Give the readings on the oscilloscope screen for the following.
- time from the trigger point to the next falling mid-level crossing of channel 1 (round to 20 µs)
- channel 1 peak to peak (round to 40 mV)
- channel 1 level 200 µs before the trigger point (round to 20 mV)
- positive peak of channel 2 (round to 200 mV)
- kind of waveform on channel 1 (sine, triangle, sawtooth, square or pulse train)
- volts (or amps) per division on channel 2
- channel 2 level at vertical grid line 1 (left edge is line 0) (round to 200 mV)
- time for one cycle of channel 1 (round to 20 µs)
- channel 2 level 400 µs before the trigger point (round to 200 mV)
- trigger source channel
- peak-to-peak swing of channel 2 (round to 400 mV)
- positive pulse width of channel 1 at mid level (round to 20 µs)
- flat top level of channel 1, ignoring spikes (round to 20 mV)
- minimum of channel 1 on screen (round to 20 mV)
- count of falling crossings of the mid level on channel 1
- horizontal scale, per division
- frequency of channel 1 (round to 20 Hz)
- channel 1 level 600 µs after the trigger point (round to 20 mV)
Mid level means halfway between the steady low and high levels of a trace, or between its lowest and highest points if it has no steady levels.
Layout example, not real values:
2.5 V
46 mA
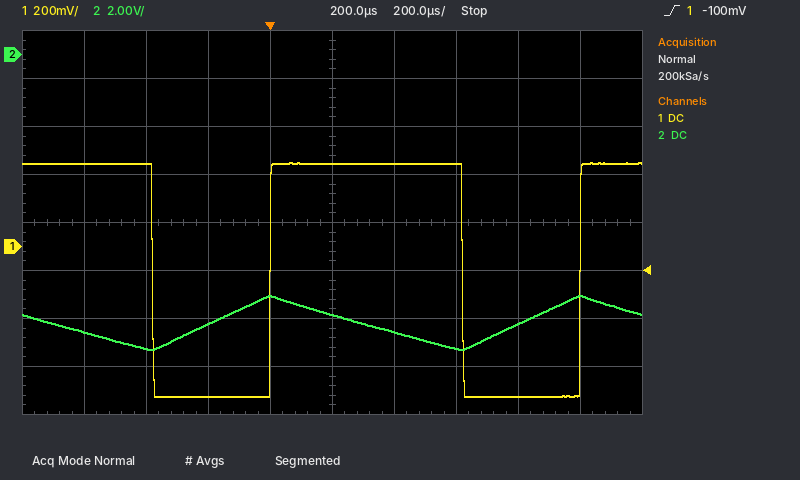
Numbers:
620 µs
960 mV
-620 mV
-10.0 V
pulse train
2 V
-11.6 V
1.00 ms
-12.2 V
channel 1
2.4 V
620 µs
340 mV
-620 mV
2
200 µs
1.00 kHz
340 mV
